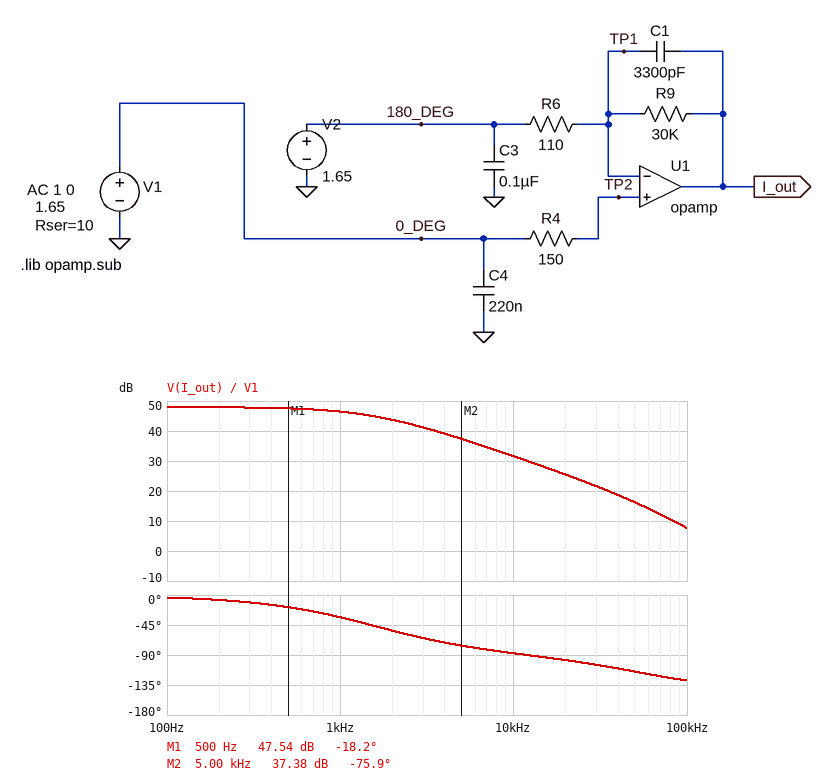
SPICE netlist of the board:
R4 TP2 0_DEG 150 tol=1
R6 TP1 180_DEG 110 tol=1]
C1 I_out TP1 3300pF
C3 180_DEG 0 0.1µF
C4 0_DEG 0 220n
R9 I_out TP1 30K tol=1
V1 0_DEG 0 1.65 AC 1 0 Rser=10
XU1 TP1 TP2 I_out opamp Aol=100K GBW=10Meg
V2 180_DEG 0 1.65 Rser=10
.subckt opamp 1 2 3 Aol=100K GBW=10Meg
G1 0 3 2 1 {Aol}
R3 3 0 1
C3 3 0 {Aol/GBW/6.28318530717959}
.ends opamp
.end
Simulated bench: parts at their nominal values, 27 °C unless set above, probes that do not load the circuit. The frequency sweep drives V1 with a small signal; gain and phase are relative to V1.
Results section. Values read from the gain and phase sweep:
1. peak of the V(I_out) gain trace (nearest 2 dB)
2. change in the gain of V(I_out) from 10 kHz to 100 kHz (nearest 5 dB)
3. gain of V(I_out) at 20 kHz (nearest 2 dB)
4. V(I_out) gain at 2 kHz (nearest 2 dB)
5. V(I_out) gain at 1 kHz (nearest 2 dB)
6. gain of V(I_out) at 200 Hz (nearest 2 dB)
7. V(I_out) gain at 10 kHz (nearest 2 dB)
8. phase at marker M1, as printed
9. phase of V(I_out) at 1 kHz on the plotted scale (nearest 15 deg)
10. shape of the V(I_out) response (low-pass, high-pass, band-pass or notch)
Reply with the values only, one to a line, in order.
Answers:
48 dB
-25 dB
26 dB
44 dB
46 dB
48 dB
32 dB
-18.2 deg
-30 deg
low-pass
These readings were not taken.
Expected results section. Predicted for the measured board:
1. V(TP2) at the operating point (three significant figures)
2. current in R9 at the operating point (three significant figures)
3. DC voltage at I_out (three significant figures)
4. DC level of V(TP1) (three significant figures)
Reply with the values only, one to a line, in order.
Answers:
1.65 V
137 nA
1.65 V
1.65 V
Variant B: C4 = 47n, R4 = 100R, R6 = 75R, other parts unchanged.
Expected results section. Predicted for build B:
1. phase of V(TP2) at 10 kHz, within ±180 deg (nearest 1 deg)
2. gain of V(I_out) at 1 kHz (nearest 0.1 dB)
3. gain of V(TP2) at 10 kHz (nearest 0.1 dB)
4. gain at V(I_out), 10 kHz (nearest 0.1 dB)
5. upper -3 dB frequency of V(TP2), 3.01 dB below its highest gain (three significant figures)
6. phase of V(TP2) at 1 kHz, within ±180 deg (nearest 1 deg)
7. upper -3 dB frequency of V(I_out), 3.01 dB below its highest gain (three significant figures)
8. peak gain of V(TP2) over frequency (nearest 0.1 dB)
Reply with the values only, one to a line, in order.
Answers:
-2 deg
49.4 dB
0 dB
34.5 dB
339 kHz
0 deg
1.53 kHz
0 dB
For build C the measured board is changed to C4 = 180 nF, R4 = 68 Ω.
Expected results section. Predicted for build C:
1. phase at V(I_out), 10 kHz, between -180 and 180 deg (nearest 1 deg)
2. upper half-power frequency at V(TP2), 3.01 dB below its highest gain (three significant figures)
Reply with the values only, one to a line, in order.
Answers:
-86 deg
88.4 kHz
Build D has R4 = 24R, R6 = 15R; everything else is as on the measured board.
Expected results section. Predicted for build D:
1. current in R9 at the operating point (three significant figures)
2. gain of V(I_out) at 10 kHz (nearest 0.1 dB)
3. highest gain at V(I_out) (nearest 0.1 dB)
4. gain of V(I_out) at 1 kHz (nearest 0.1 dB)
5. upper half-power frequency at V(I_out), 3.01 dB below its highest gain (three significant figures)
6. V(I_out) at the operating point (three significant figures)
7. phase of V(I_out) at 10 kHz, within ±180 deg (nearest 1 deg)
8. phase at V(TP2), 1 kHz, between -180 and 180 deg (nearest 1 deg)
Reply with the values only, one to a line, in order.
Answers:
652 nA
44.0 dB
61.5 dB
59.6 dB
1.36 kHz
1.63 V
-89 deg
-1 deg
